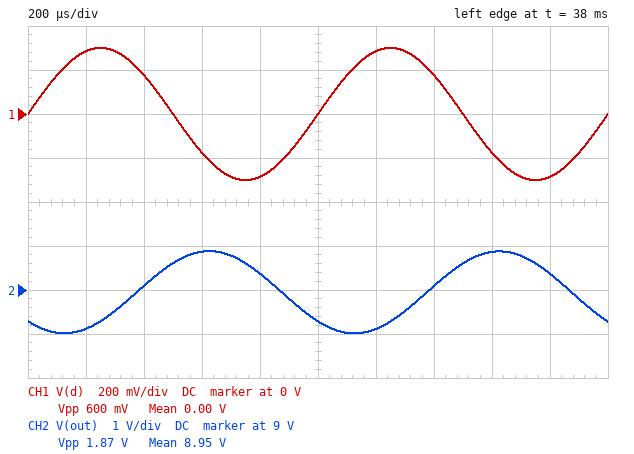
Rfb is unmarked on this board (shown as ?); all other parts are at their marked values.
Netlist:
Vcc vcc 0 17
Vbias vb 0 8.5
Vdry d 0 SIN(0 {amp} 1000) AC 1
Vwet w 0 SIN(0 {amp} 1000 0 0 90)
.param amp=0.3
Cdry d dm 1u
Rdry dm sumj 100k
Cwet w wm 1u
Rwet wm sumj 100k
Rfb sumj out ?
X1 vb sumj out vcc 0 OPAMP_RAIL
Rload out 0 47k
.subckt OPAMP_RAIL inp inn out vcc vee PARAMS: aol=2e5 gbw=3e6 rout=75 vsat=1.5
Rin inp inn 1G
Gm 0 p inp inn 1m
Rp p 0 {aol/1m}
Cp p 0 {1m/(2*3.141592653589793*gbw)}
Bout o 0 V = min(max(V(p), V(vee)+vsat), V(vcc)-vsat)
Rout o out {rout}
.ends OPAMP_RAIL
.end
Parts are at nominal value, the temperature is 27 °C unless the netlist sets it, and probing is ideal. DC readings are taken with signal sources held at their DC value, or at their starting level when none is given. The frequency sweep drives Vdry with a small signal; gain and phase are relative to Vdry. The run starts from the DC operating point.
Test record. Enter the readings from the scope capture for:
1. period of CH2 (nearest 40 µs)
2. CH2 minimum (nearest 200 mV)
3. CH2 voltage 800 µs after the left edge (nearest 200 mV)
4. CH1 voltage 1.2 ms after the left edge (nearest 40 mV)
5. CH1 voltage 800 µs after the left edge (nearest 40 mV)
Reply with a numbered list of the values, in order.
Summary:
1. 1.00 ms
2. 8.0 V
3. 9.4 V
4. 280 mV
5. -280 mV
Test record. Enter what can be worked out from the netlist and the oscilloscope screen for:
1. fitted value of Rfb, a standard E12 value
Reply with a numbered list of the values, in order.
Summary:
1. 220 kΩ
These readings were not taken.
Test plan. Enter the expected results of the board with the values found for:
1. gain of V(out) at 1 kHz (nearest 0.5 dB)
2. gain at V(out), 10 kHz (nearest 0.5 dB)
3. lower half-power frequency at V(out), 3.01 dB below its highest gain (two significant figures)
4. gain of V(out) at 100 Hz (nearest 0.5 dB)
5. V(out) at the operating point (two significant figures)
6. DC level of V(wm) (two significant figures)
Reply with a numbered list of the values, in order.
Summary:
1. 7.0 dB
2. 7.0 dB
3. 1.6 Hz
4. 7.0 dB
5. 8.5 V
6. 8.5 V
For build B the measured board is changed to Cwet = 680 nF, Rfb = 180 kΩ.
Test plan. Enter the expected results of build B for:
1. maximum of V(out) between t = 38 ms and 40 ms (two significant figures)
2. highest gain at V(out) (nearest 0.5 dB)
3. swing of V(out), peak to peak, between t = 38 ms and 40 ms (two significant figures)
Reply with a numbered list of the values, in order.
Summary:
1. 9.6 V
2. 5.0 dB
3. 1.5 V
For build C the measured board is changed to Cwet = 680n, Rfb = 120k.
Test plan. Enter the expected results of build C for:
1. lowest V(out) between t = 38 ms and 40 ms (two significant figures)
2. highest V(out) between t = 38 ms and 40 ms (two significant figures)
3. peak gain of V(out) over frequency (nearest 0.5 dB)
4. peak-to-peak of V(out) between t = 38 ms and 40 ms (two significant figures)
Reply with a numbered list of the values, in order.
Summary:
1. 8.2 V
2. 9.2 V
3. 1.5 dB
4. 1.0 V
